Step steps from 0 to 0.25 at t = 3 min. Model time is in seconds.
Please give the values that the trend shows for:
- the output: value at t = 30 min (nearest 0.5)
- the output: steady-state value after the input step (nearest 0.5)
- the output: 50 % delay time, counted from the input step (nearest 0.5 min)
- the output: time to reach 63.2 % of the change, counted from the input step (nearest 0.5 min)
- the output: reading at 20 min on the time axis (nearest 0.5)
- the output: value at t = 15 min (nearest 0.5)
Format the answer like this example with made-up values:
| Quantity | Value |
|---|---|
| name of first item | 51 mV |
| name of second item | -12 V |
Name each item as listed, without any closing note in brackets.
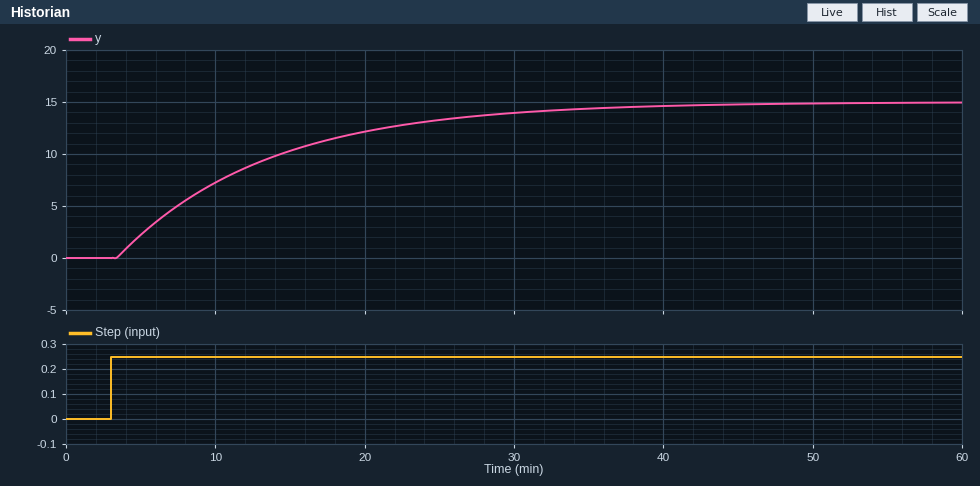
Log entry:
| Quantity | Value |
|---|---|
| the output: value at t = 30 min | 14.0 |
| the output: steady-state value after the input step | 15.0 |
| the output: 50 % delay time, counted from the input step | 7.5 min |
| the output: time to reach 63.2 % of the change, counted from the input step | 10.5 min |
| the output: reading at 20 min on the time axis | 12.0 |
| the output: value at t = 15 min | 10.5 |
